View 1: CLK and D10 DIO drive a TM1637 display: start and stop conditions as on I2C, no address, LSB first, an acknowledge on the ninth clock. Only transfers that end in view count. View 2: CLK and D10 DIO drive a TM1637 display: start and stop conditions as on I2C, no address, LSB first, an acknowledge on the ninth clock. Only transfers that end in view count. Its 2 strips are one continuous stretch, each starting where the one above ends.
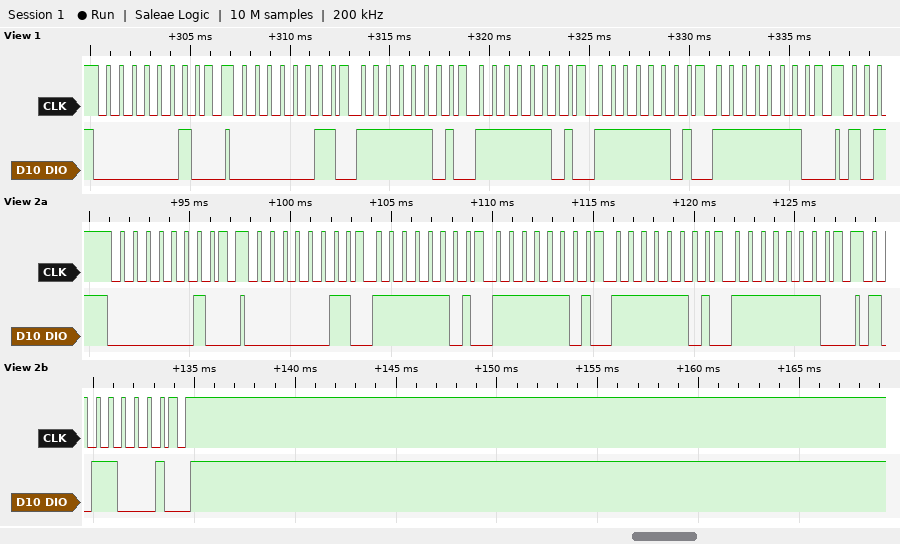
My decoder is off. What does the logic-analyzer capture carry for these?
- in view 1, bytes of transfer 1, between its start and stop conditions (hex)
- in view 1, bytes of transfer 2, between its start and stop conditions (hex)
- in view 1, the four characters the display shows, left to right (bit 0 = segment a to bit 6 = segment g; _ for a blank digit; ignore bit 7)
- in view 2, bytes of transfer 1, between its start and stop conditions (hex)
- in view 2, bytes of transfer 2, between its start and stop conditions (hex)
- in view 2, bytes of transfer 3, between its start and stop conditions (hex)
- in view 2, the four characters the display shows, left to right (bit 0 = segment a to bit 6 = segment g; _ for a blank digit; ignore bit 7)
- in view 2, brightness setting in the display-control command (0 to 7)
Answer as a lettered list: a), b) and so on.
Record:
a) 40
b) C0 BF BF BF 7F
c) 0008
d) 40
e) C0 BF BF BF 7F
f) 8D
g) 0008
h) 5
